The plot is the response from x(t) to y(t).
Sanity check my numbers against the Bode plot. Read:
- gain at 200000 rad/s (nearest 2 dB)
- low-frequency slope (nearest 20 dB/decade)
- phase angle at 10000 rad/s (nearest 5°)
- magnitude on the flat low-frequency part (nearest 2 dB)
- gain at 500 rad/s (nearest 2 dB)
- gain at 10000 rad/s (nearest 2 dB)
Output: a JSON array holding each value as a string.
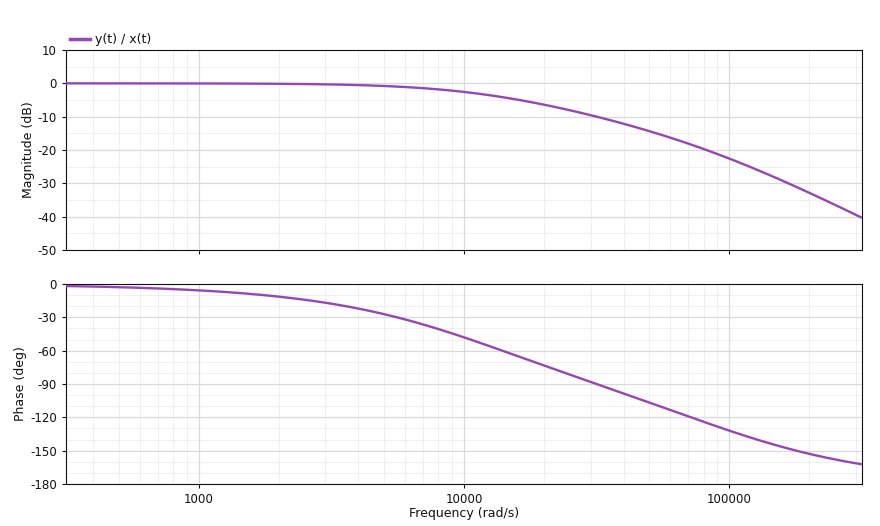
["-32 dB", "0 dB/decade", "-50°", "0 dB", "0 dB", "-2 dB"]
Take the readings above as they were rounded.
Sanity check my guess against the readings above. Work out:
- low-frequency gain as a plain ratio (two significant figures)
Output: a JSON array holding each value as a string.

["1.0"]
